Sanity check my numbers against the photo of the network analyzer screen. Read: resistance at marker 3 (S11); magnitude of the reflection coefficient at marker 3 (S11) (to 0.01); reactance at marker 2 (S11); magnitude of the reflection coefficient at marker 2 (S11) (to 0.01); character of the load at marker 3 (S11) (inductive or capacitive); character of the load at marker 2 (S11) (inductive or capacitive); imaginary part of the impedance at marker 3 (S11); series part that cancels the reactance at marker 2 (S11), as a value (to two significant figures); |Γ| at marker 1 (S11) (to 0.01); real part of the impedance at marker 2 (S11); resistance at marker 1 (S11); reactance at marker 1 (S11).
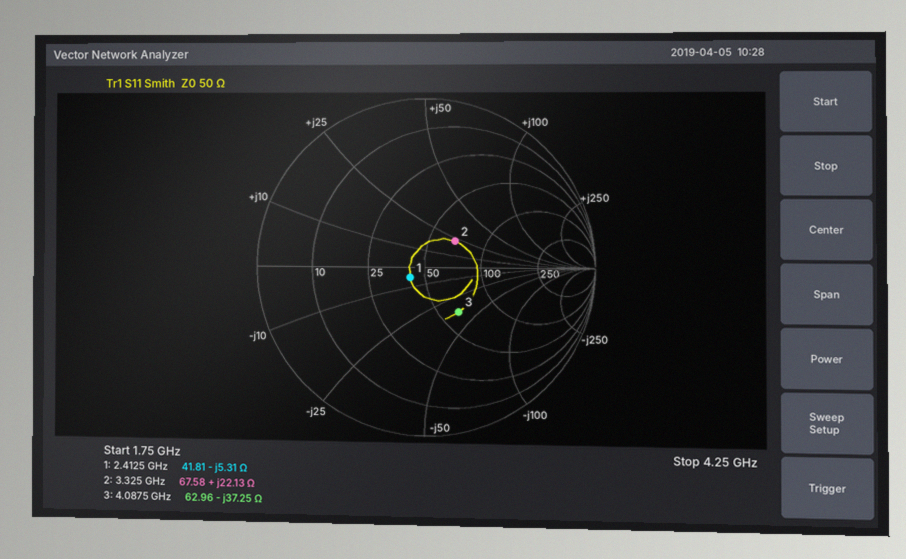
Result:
62.96 Ω
0.33
+22.13 Ω
0.24
capacitive
inductive
-37.25 Ω
2.2 pF
0.11
67.58 Ω
41.81 Ω
-5.31 Ω
